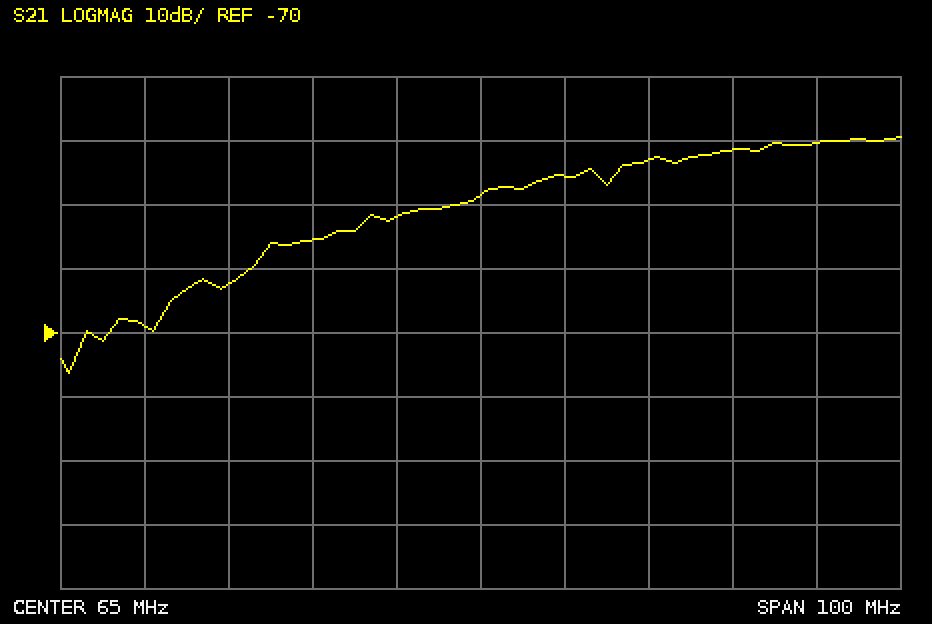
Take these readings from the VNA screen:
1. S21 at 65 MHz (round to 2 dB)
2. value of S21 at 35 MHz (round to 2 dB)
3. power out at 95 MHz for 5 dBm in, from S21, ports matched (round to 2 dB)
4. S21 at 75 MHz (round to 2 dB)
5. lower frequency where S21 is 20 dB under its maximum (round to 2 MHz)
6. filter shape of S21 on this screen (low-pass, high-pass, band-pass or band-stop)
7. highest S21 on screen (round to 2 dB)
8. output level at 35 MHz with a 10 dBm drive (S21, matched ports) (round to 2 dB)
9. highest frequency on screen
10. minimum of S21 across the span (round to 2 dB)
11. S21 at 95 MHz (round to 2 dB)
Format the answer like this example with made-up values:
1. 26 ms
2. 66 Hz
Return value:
1. -48 dB
2. -62 dB
3. -36 dBm
4. -46 dB
5. 38 MHz
6. high-pass
7. -40 dB
8. -52 dBm
9. 115 MHz
10. -76 dB
11. -42 dB
